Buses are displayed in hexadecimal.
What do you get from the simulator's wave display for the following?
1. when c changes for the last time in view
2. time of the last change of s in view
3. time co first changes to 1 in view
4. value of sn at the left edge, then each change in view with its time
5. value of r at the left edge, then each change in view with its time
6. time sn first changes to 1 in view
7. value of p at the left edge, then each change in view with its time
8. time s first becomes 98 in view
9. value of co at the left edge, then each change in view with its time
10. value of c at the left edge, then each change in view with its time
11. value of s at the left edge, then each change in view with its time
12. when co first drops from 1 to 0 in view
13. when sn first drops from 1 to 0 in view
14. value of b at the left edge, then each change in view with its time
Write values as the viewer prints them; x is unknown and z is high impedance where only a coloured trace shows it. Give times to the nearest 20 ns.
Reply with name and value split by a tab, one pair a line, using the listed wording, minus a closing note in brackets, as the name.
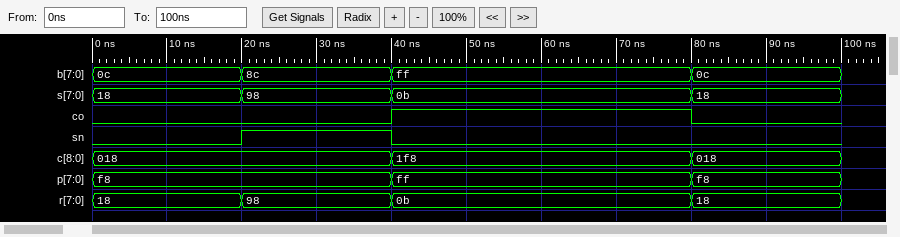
when c changes for the last time in view	80 ns
time of the last change of s in view	80 ns
time co first changes to 1 in view	40 ns
value of sn at the left edge, then each change in view with its time	0, 1 at 20 ns, 0 at 40 ns
value of r at the left edge, then each change in view with its time	18, 98 at 20 ns, 0b at 40 ns, 18 at 80 ns
time sn first changes to 1 in view	20 ns
value of p at the left edge, then each change in view with its time	f8, ff at 40 ns, f8 at 80 ns
time s first becomes 98 in view	20 ns
value of co at the left edge, then each change in view with its time	0, 1 at 40 ns, 0 at 80 ns
value of c at the left edge, then each change in view with its time	018, 1f8 at 40 ns, 018 at 80 ns
value of s at the left edge, then each change in view with its time	18, 98 at 20 ns, 0b at 40 ns, 18 at 80 ns
when co first drops from 1 to 0 in view	80 ns
when sn first drops from 1 to 0 in view	40 ns
value of b at the left edge, then each change in view with its time	0c, 8c at 20 ns, ff at 40 ns, 0c at 80 ns
